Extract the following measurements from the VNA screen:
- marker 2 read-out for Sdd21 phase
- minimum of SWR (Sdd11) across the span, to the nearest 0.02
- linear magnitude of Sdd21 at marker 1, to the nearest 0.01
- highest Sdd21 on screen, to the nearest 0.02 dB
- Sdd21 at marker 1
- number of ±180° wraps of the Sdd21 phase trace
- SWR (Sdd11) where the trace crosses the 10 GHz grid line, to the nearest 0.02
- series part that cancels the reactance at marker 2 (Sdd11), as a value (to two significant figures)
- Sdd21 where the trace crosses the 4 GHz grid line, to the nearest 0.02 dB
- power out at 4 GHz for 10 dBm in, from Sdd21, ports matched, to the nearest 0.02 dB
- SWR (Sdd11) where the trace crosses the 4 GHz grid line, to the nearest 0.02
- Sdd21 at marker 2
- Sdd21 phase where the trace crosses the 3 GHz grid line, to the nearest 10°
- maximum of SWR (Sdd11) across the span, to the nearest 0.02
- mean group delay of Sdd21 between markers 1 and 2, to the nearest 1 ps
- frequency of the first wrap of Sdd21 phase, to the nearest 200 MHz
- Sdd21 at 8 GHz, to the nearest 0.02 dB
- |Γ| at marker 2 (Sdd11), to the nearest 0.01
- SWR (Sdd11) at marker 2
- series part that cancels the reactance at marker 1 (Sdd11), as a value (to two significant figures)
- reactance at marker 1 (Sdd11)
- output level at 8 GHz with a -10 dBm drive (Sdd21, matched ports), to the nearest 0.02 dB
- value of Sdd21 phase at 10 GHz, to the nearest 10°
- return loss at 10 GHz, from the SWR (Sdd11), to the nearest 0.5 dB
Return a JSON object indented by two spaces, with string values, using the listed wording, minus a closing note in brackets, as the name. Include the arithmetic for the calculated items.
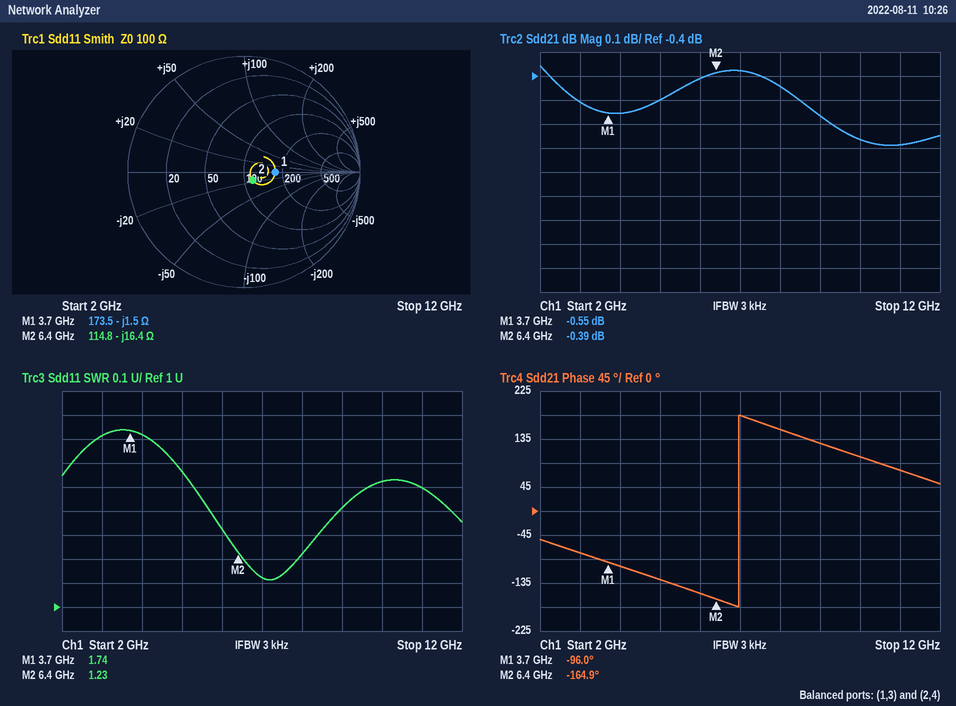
{
  "marker 2 read-out for Sdd21 phase": "-164.9°",
  "minimum of SWR (Sdd11) across the span, to the nearest 0.02": "1.12",
  "linear magnitude of Sdd21 at marker 1, to the nearest 0.01": "10^(-0.55/20) ≈ 0.94",
  "highest Sdd21 on screen, to the nearest 0.02 dB": "-0.36 dB",
  "Sdd21 at marker 1": "-0.55 dB",
  "number of ±180° wraps of the Sdd21 phase trace": "1",
  "SWR (Sdd11) where the trace crosses the 10 GHz grid line, to the nearest 0.02": "1.52",
  "series part that cancels the reactance at marker 2 (Sdd11), as a value": "L = 16.4 Ω/(2π × 6.4 GHz) ≈ 408 pH, so 410 pH to two significant figures",
  "Sdd21 where the trace crosses the 4 GHz grid line, to the nearest 0.02 dB": "-0.56 dB",
  "power out at 4 GHz for 10 dBm in, from Sdd21, ports matched, to the nearest 0.02 dB": "10 dBm + (-0.56 dB) = 9.44 dBm",
  "SWR (Sdd11) where the trace crosses the 4 GHz grid line, to the nearest 0.02": "1.72",
  "Sdd21 at marker 2": "-0.39 dB",
  "Sdd21 phase where the trace crosses the 3 GHz grid line, to the nearest 10°": "-80°",
  "maximum of SWR (Sdd11) across the span, to the nearest 0.02": "1.74",
  "mean group delay of Sdd21 between markers 1 and 2, to the nearest 1 ps": "−(-164.9° − (-96°))/(360° × 2.7 GHz) ≈ 71 ps",
  "frequency of the first wrap of Sdd21 phase, to the nearest 200 MHz": "7.0 GHz",
  "Sdd21 at 8 GHz, to the nearest 0.02 dB": "-0.44 dB",
  "|Γ| at marker 2 (Sdd11), to the nearest 0.01": "0.10",
  "SWR (Sdd11) at marker 2": "1.23",
  "series part that cancels the reactance at marker 1 (Sdd11), as a value": "L = 1.5 Ω/(2π × 3.7 GHz) ≈ 65 pH",
  "reactance at marker 1": "-1.5 Ω",
  "output level at 8 GHz with a -10 dBm drive (Sdd21, matched ports), to the nearest 0.02 dB": "-10 dBm + (-0.44 dB) = -10.44 dBm",
  "value of Sdd21 phase at 10 GHz, to the nearest 10°": "100°",
  "return loss at 10 GHz, from the SWR (Sdd11), to the nearest 0.5 dB": "−20 log10((1.52 − 1)/(1.52 + 1)) ≈ 13.7 dB, so 13.5 dB to the nearest 0.5 dB"
}
